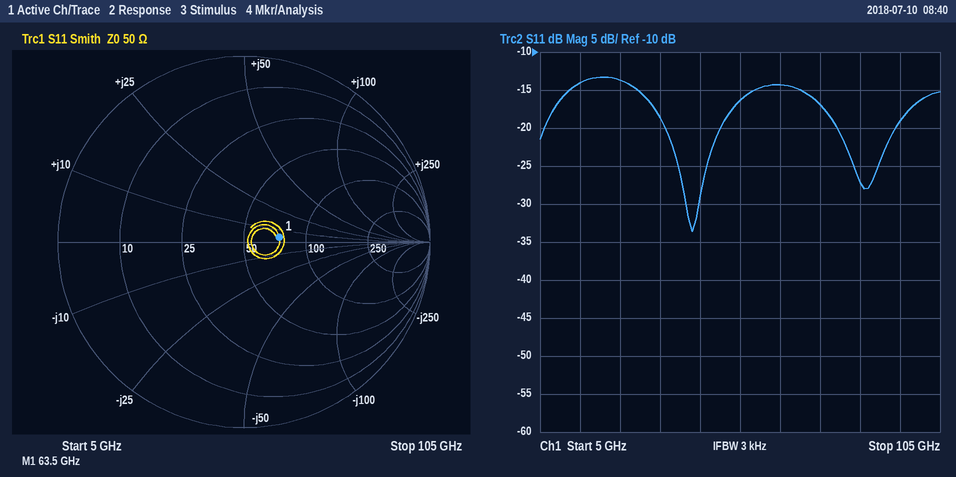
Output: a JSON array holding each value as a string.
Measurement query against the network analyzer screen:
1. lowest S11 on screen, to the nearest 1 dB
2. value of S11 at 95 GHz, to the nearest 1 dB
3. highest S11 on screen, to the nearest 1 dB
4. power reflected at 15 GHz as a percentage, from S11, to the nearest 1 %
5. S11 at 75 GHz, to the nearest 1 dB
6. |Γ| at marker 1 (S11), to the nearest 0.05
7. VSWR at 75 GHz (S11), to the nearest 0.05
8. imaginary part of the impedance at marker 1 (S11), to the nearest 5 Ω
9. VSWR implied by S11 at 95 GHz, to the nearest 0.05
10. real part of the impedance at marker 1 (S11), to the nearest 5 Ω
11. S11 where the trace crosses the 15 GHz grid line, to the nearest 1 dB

["-34 dB", "-19 dB", "-13 dB", "4 %", "-17 dB", "0.20", "1.35", "+5 Ω", "1.25", "75 Ω", "-14 dB"]
